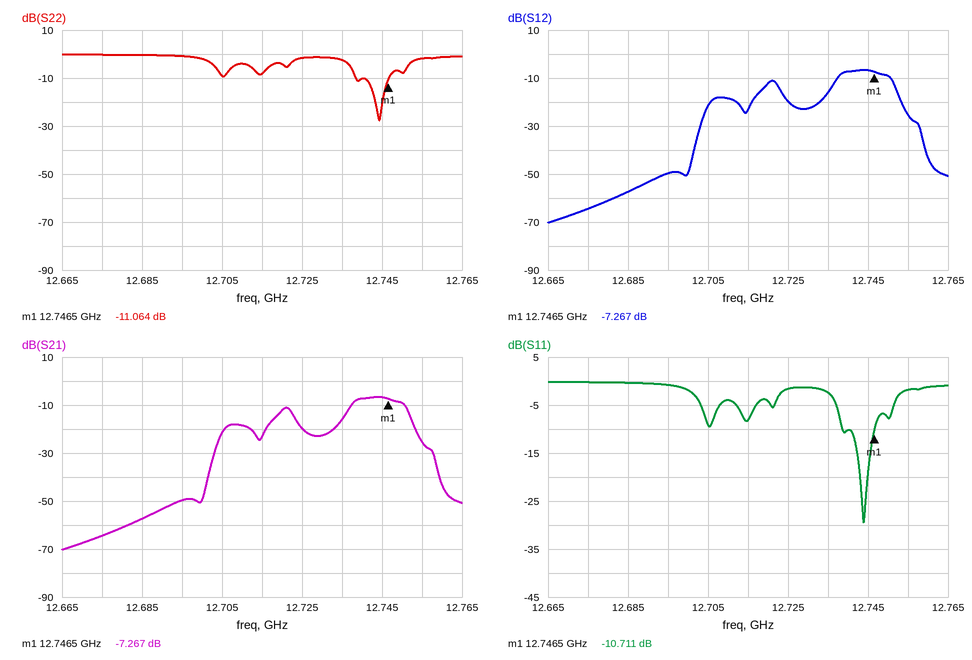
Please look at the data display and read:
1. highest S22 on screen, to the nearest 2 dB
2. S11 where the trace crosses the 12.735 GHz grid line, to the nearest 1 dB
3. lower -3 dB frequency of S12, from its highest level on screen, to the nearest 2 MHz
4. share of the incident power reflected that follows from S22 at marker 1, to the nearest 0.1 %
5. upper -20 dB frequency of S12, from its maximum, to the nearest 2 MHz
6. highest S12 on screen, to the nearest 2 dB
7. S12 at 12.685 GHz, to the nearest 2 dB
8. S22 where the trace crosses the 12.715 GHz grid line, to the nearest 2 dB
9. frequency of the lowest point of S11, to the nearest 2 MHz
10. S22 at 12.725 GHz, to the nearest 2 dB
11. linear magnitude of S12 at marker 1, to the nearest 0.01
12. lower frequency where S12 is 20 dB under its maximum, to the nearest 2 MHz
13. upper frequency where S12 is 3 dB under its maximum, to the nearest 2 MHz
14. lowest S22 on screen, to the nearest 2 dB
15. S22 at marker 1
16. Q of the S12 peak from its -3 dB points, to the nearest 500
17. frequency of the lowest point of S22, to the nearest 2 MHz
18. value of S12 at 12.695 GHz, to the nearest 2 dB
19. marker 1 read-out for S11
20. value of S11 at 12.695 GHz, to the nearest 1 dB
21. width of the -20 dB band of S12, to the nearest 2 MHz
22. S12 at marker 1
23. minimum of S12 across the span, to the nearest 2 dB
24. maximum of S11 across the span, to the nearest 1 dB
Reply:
0 dB
-2 dB
12.738 GHz
7.8 %
12.756 GHz
-6 dB
-58 dB
-8 dB
12.744 GHz
-2 dB
0.43
12.704 GHz
12.750 GHz
-28 dB
-11.064 dB
1000
12.744 GHz
-50 dB
-10.711 dB
-1 dB
52 MHz
-7.267 dB
-70 dB
0 dB
